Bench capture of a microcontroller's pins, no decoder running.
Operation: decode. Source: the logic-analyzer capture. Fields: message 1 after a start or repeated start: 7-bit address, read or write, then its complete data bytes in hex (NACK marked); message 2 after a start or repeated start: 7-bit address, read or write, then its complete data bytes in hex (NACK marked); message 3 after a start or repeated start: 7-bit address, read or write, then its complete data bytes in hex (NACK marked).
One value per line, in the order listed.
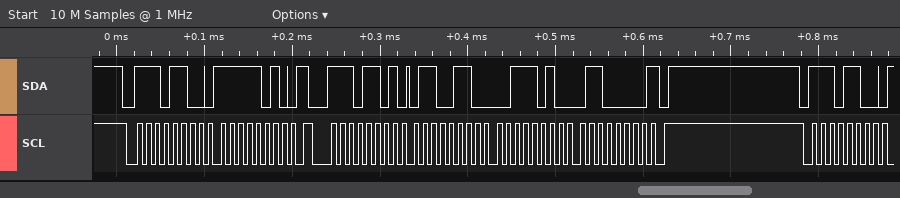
0x76 write: FA
0x76 read: 66 3A 60 NACK
0x76 write
